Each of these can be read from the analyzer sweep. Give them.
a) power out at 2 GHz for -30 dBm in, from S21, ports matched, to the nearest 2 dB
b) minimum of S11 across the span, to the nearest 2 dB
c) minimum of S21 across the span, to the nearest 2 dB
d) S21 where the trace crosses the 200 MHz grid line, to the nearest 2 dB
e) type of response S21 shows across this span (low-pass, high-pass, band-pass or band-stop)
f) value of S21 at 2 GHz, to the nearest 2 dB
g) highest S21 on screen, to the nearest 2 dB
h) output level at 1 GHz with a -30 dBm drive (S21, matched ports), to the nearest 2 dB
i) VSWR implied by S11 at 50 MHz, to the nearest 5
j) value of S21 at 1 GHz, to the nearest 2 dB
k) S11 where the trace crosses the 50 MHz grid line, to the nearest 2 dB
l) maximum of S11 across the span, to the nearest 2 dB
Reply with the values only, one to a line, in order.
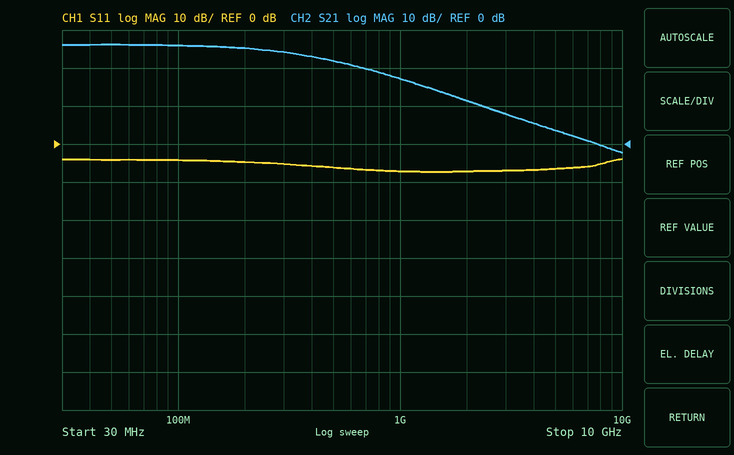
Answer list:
-18 dBm
-8 dB
-2 dB
26 dB
low-pass
12 dB
26 dB
-12 dBm
5
18 dB
-4 dB
-4 dB
